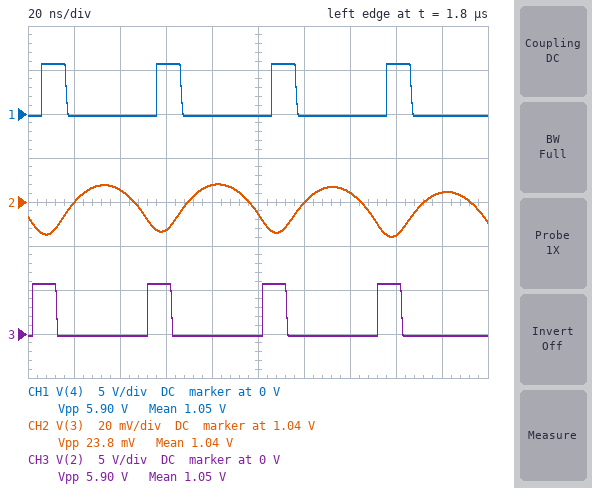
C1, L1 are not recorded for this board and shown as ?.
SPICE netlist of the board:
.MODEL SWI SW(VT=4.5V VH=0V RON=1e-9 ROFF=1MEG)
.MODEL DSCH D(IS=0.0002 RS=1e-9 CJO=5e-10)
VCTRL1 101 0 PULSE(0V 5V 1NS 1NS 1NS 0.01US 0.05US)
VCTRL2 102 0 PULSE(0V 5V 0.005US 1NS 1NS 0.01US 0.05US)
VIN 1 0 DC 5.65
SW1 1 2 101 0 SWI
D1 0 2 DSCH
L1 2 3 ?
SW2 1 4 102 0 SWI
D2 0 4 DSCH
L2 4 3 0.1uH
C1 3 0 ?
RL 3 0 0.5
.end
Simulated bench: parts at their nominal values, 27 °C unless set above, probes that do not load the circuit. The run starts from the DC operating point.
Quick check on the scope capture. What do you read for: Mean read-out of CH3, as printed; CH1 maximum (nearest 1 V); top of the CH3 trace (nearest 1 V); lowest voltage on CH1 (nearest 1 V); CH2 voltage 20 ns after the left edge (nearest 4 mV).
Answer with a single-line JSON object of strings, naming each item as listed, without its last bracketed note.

{"Mean read-out of CH3, as printed": "1.05 V", "CH1 maximum": "6 V", "top of the CH3 trace": "6 V", "lowest voltage on CH1": "0 V", "CH2 voltage 20 ns after the left edge": "1.040 V"}
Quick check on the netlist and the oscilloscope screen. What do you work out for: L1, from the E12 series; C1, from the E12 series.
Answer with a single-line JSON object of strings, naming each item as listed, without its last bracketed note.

{"L1, from the E12 series": "33 nH", "C1, from the E12 series": "560 nF"}
